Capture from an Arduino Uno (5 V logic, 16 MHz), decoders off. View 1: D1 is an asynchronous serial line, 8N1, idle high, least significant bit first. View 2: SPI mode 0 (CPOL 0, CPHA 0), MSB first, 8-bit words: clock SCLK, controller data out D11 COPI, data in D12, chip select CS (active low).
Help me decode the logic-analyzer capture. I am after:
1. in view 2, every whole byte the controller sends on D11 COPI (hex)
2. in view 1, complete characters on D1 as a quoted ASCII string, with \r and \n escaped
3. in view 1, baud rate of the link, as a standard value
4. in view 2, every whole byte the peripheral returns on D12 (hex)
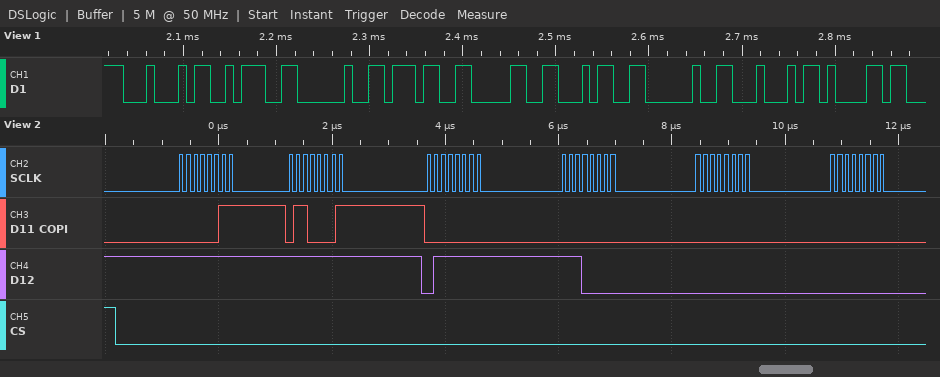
03 61 00 00 00 00
"D: 704 Da"
115200 baud
FF FF 7F E0 00 00
